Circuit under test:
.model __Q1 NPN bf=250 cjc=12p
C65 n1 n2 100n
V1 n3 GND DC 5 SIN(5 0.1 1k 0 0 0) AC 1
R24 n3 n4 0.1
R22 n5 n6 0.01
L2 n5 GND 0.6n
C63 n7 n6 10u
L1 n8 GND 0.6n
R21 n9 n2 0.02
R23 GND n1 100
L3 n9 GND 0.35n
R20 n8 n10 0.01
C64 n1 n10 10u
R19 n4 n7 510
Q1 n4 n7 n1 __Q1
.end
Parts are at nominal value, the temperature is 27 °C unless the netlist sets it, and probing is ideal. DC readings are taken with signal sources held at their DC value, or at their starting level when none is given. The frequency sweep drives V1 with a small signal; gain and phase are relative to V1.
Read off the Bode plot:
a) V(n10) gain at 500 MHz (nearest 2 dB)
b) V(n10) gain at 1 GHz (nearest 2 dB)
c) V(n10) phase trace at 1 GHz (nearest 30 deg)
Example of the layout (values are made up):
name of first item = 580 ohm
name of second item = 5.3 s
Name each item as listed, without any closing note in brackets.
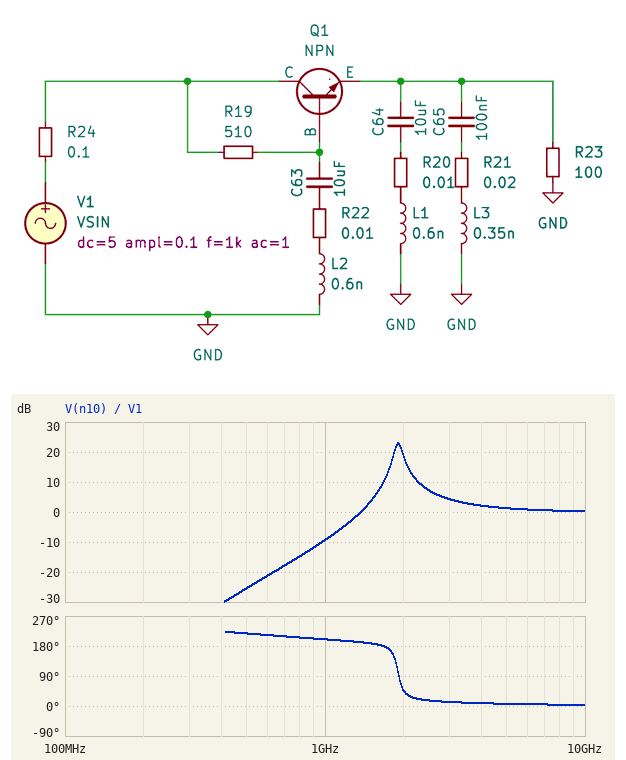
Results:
V(n10) gain at 500 MHz = -26 dB
V(n10) gain at 1 GHz = -10 dB
V(n10) phase trace at 1 GHz = 210 deg
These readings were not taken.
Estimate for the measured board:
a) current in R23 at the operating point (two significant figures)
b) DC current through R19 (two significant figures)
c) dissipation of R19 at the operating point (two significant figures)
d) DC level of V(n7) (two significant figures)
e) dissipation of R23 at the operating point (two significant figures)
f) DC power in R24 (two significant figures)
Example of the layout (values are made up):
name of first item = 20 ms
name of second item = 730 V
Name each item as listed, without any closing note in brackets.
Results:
current in R23 at the operating point = 40 mA
DC current through R19 = 160 µA
dissipation of R19 at the operating point = 13 µW
DC level of V(n7) = 4.9 V
dissipation of R23 at the operating point = 160 mW
DC power in R24 = 160 µW
